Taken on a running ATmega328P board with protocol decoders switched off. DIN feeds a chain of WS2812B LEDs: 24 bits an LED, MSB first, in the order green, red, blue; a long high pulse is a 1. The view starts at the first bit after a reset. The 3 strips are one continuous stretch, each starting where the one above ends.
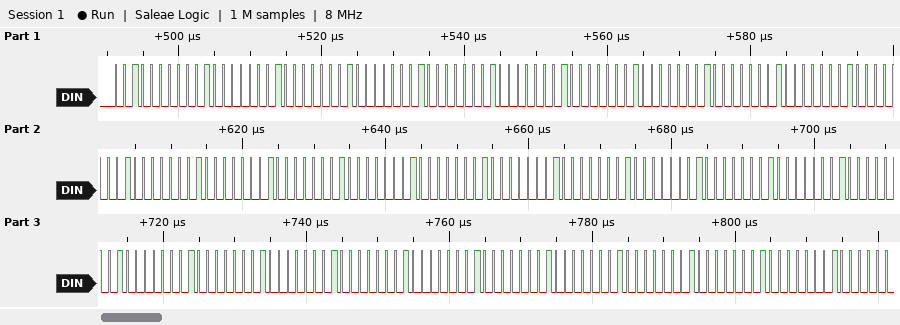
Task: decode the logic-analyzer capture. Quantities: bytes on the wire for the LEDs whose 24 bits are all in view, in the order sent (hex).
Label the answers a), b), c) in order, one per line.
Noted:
a) 20 20 20 20 20 20 20 20 20 20 20 20 20 20 20 20 20 20 20 20 20 20 20 20 20 20 20 20 20 20 20 20 20
